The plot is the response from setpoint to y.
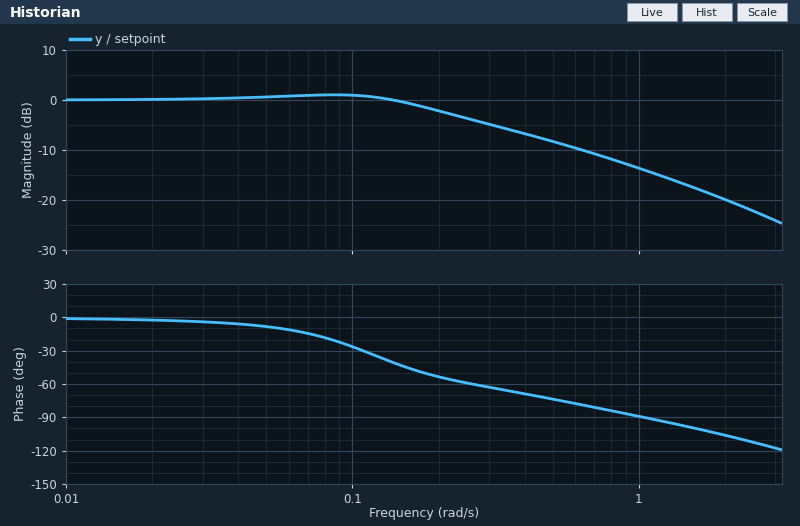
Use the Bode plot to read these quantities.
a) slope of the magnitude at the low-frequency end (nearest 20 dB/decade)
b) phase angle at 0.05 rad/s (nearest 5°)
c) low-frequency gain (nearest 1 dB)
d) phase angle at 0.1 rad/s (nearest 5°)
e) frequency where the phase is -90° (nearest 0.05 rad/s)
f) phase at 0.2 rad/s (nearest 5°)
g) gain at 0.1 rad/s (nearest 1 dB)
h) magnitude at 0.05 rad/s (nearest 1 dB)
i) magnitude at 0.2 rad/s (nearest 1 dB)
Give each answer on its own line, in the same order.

0 dB/decade
-10°
0 dB
-25°
1.05 rad/s
-55°
1 dB
1 dB
-2 dB
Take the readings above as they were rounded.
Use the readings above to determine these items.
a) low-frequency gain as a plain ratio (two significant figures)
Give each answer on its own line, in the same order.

1.0
